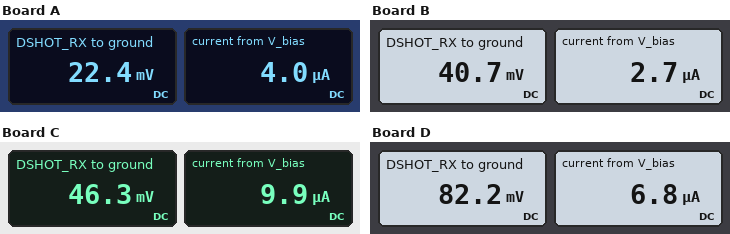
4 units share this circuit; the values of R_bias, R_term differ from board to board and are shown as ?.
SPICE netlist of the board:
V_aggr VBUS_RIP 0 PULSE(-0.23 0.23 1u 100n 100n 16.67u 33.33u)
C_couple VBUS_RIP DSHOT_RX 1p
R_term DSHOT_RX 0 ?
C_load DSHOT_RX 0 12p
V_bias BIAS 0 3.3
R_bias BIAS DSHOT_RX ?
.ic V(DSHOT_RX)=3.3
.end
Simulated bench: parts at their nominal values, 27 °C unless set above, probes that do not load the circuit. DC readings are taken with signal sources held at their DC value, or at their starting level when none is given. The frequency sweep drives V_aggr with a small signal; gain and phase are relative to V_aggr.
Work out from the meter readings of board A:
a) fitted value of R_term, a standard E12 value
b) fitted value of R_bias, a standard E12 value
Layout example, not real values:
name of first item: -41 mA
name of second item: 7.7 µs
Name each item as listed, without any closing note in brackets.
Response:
fitted value of R_term, a standard E12 value: 5.6 kΩ
fitted value of R_bias, a standard E12 value: 820 kΩ
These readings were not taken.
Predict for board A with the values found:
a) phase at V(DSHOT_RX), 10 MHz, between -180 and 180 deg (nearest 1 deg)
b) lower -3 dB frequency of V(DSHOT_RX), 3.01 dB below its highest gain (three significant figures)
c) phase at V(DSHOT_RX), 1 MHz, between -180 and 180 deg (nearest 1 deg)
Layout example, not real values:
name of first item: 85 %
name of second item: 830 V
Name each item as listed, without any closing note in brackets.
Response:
phase at V(DSHOT_RX), 10 MHz, between -180 and 180 deg: 12 deg
lower -3 dB frequency of V(DSHOT_RX), 3.01 dB below its highest gain: 2.20 MHz
phase at V(DSHOT_RX), 1 MHz, between -180 and 180 deg: 66 deg
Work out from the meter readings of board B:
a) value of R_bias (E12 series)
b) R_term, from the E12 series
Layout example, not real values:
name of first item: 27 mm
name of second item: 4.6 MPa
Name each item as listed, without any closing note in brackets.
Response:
value of R_bias: 1.2 MΩ
R_term, from the E12 series: 15 kΩ
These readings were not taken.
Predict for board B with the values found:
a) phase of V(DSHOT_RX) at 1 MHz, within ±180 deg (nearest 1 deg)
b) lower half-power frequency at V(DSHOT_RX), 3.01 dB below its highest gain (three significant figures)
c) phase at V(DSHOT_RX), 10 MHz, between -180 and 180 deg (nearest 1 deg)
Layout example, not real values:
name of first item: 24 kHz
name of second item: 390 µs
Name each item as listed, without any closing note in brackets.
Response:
phase of V(DSHOT_RX) at 1 MHz, within ±180 deg: 40 deg
lower half-power frequency at V(DSHOT_RX), 3.01 dB below its highest gain: 826 kHz
phase at V(DSHOT_RX), 10 MHz, between -180 and 180 deg: 5 deg
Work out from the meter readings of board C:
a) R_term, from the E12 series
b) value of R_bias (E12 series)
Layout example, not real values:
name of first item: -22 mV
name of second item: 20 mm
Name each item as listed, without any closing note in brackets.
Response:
R_term, from the E12 series: 4.7 kΩ
value of R_bias: 330 kΩ
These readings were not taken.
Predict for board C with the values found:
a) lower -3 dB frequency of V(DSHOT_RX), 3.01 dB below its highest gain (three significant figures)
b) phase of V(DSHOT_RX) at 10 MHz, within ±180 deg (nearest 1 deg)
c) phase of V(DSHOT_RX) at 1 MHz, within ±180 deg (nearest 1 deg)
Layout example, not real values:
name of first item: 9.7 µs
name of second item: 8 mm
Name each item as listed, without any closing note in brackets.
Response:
lower -3 dB frequency of V(DSHOT_RX), 3.01 dB below its highest gain: 2.64 MHz
phase of V(DSHOT_RX) at 10 MHz, within ±180 deg: 15 deg
phase of V(DSHOT_RX) at 1 MHz, within ±180 deg: 69 deg
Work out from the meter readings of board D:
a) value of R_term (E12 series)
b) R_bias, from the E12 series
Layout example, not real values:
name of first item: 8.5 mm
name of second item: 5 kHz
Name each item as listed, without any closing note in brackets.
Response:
value of R_term: 12 kΩ
R_bias, from the E12 series: 470 kΩ
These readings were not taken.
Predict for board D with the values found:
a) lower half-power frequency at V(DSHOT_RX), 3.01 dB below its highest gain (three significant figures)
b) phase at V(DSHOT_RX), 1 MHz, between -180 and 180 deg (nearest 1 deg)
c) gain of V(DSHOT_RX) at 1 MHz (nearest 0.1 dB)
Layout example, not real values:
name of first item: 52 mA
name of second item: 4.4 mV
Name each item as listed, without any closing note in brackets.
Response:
lower half-power frequency at V(DSHOT_RX), 3.01 dB below its highest gain: 1.05 MHz
phase at V(DSHOT_RX), 1 MHz, between -180 and 180 deg: 46 deg
gain of V(DSHOT_RX) at 1 MHz: -25.5 dB
